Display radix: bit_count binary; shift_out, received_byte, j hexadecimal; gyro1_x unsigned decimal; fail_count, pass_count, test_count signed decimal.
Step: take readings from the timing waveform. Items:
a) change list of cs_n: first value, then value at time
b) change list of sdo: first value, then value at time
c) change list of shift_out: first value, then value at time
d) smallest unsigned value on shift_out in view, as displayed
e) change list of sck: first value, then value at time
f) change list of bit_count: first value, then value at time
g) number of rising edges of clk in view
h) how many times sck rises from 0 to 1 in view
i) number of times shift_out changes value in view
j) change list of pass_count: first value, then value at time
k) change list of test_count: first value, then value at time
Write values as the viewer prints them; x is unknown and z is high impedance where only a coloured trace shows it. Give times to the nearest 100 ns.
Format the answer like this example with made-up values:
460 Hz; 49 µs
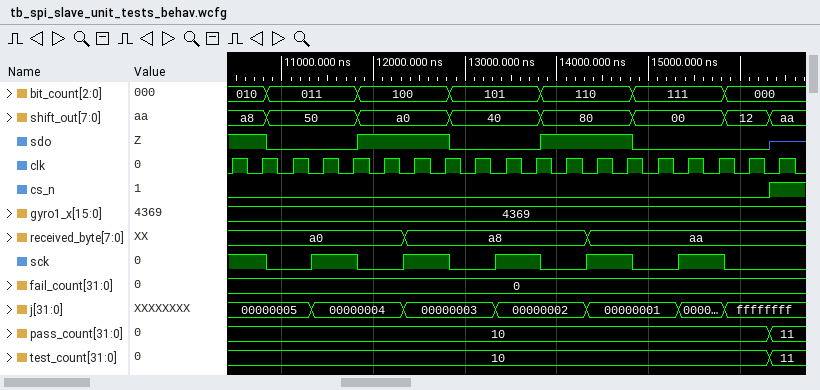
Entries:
0, 1 at 16300 ns; 1, 0 at 10800 ns, 1 at 11800 ns, 0 at 12800 ns, 1 at 13800 ns, 0 at 14800 ns, z at 16300 ns; a8, 50 at 10800 ns, a0 at 11800 ns, 40 at 12800 ns, 80 at 13800 ns, 00 at 14800 ns, 12 at 15800 ns, aa at 16300 ns; 00; 1, 0 at 10800 ns, 1 at 11300 ns, 0 at 11800 ns, 1 at 12300 ns, 0 at 12800 ns, 1 at 13300 ns, 0 at 13800 ns, 1 at 14300 ns, 0 at 14800 ns, 1 at 15300 ns, 0 at 15800 ns; 010, 011 at 10800 ns, 100 at 11800 ns, 101 at 12800 ns, 110 at 13800 ns, 111 at 14800 ns, 000 at 15800 ns; 19; 5; 7; 10, 11 at 16300 ns; 10, 11 at 16300 ns
